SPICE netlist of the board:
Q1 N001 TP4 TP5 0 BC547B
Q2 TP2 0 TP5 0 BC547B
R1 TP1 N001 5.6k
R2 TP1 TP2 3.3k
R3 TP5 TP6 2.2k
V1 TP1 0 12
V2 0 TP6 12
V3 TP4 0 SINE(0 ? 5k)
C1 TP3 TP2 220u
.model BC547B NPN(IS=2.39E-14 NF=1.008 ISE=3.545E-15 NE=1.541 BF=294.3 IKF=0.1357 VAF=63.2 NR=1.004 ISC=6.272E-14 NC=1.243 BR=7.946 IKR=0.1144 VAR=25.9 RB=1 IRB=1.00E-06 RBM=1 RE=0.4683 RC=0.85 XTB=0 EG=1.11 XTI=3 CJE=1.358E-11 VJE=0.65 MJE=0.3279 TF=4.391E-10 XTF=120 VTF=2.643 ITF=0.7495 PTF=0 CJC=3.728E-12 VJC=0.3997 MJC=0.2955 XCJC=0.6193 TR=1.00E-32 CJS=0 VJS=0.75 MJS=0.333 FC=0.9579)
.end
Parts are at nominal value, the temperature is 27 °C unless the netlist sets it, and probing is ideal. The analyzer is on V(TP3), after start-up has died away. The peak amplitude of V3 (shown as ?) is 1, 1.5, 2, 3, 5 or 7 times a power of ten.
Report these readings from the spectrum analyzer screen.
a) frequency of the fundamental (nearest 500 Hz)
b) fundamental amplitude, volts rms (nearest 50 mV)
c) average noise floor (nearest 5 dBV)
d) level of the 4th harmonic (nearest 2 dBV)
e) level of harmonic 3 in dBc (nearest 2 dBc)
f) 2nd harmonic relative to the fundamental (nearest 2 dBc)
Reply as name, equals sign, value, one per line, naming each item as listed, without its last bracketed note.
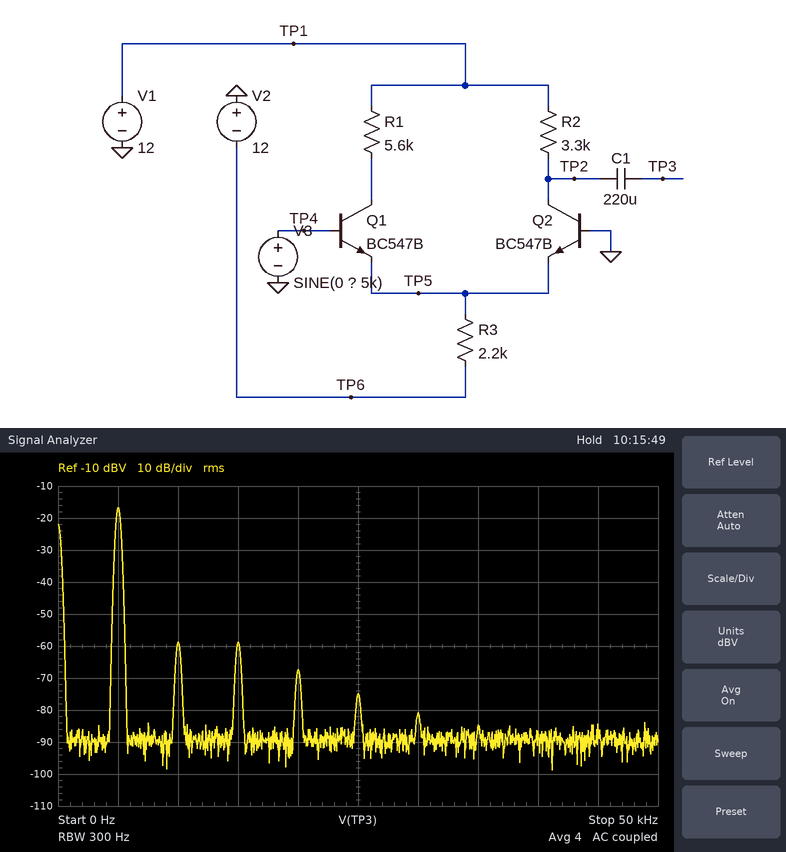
frequency of the fundamental = 5.0 kHz
fundamental amplitude, volts rms = 150 mV
average noise floor = -90 dBV
level of the 4th harmonic = -68 dBV
level of harmonic 3 in dBc = -42 dBc
2nd harmonic relative to the fundamental = -42 dBc
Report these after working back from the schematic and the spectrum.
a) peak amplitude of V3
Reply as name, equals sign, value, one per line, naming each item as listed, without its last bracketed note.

peak amplitude of V3 = 5 mV
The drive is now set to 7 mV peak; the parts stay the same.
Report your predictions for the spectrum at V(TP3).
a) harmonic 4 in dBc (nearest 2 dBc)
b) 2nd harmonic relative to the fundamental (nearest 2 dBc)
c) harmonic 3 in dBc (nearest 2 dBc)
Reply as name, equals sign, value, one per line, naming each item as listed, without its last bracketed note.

harmonic 4 in dBc = -28 dBc
2nd harmonic relative to the fundamental = -24 dBc
harmonic 3 in dBc = -24 dBc
